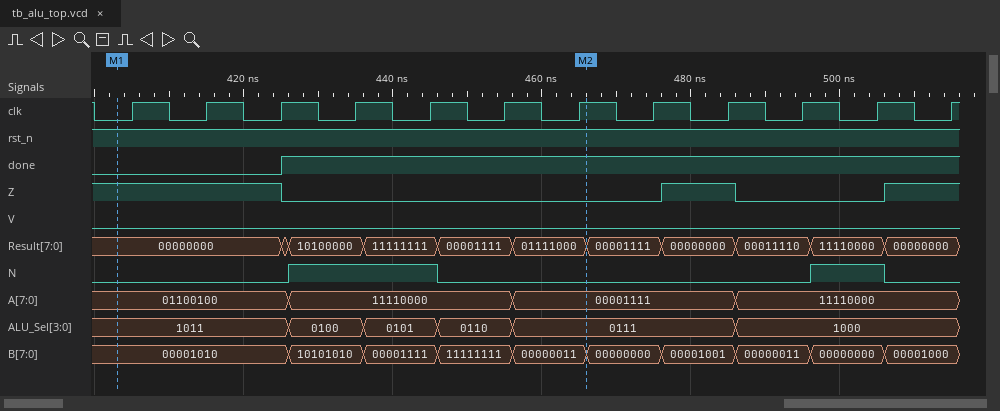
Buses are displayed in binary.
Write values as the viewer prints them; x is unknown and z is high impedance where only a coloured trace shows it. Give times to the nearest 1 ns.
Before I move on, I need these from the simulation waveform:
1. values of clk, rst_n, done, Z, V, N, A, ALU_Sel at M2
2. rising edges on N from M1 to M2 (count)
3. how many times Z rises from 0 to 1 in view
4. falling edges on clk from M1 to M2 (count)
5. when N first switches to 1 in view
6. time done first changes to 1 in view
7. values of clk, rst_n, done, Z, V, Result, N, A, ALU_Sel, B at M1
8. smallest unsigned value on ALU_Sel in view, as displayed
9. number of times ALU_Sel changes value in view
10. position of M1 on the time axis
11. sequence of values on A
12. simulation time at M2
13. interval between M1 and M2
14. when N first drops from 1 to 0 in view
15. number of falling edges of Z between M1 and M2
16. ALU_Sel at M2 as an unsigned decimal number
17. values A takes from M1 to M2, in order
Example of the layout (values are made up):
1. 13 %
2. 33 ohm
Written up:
1. clk=1, rst_n=1, done=1, Z=0, V=0, N=0, A=00001111, ALU_Sel=0111
2. 1
3. 2
4. 6
5. 426 ns
6. 425 ns
7. clk=0, rst_n=1, done=0, Z=1, V=0, Result=00000000, N=0, A=01100100, ALU_Sel=1011, B=00001010
8. 0100
9. 5
10. 403 ns
11. 01100100, 11110000, 00001111, 11110000
12. 466 ns
13. 63 ns
14. 446 ns
15. 1
16. 7
17. 01100100, 11110000, 00001111
